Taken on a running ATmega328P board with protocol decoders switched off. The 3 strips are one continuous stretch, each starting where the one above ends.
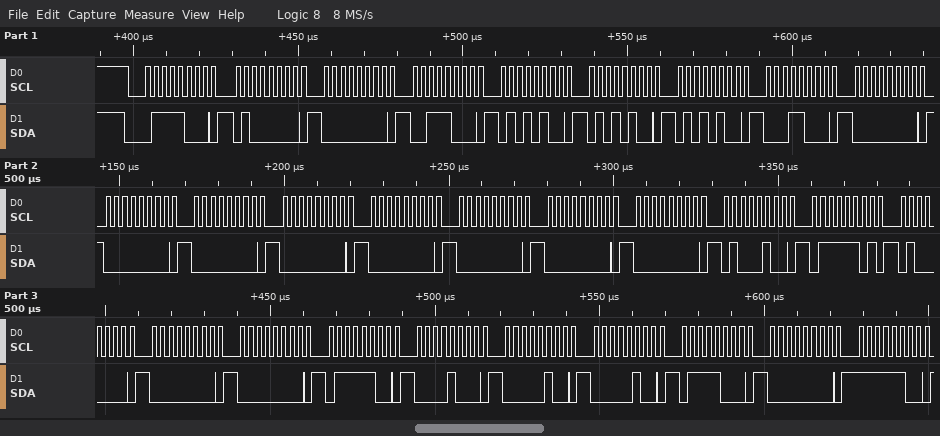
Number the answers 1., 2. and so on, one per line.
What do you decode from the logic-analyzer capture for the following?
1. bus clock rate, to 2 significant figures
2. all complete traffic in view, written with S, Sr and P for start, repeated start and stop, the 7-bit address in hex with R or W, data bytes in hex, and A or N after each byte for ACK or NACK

1. 400 kHz
2. S 3CW A 40 A 00 A 38 A 54 A 54 A 54 A 18 A 00 A 00 A 00 A 00 A 00 A 00 A 00 A 00 A 44 A 7D A 40 A 00 A 00 A 7C A 08 A 04 A 04 A 78 A 00 A FC A
